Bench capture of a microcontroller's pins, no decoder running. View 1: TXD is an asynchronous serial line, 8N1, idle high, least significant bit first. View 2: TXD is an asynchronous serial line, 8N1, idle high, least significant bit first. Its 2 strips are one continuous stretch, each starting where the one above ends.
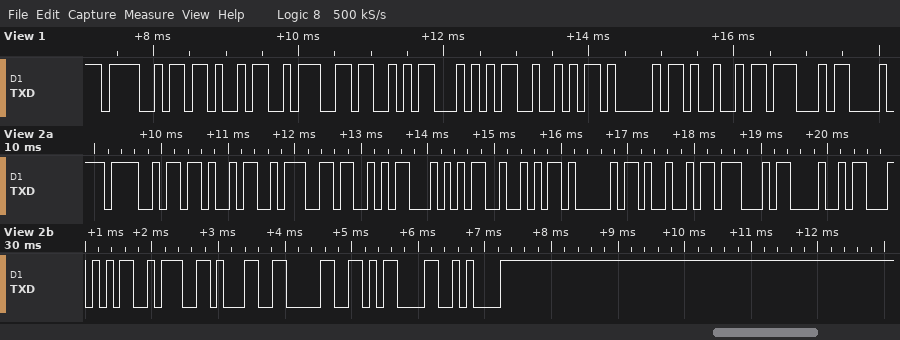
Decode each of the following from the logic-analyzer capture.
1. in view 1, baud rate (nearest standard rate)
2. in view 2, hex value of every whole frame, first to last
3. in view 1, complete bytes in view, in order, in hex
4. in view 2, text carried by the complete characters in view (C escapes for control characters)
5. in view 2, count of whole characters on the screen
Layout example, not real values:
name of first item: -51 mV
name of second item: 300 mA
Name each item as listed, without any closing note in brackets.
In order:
in view 1, baud rate: 9600 baud
in view 2, hex value of every whole frame, first to last: 4F 4B 3A 53 54 52 41 49 47 48 54 3A 31 30 0D 0A
in view 1, complete bytes in view, in order, in hex: 4F 4B 3A 53 54 52 41 49 47
in view 2, text carried by the complete characters in view: "OK:STRAIGHT:10\r\n"
in view 2, count of whole characters on the screen: 16
